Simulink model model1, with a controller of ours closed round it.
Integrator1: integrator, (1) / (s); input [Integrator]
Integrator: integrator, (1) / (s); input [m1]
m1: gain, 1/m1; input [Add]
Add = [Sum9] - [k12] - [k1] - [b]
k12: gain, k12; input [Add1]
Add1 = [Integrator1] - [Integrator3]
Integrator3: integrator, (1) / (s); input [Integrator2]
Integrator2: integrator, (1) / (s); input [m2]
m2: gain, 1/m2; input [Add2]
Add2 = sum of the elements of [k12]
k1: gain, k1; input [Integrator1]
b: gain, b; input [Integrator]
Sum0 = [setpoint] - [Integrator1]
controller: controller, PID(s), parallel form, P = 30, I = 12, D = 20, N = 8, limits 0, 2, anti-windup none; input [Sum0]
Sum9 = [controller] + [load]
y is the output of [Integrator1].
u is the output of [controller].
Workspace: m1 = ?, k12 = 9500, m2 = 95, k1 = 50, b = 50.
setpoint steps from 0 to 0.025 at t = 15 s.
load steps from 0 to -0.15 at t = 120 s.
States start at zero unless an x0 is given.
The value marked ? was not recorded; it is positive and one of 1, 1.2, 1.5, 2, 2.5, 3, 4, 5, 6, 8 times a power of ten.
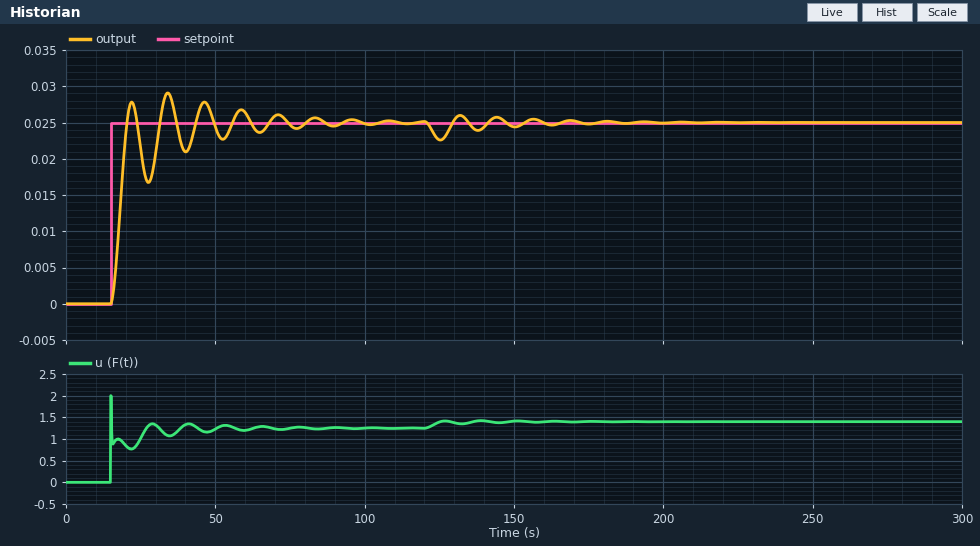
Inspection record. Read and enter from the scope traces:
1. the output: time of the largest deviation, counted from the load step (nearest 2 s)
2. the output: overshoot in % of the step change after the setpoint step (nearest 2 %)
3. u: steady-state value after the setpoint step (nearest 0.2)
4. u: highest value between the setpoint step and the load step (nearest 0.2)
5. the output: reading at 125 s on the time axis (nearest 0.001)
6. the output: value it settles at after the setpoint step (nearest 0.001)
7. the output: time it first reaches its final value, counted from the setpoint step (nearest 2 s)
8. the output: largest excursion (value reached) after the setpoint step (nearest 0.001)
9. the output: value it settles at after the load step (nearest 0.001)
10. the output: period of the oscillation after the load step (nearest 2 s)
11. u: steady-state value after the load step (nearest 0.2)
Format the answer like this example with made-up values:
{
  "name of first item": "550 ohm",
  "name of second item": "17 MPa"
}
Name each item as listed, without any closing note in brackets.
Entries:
{
  "the output: time of the largest deviation, counted from the load step": "6 s",
  "the output: overshoot in % of the step change after the setpoint step": "16 %",
  "u: steady-state value after the setpoint step": "1.2",
  "u: highest value between the setpoint step and the load step": "2.0",
  "the output: reading at 125 s on the time axis": "0.023",
  "the output: value it settles at after the setpoint step": "0.025",
  "the output: time it first reaches its final value, counted from the setpoint step": "6 s",
  "the output: largest excursion (value reached) after the setpoint step": "0.029",
  "the output: value it settles at after the load step": "0.025",
  "the output: period of the oscillation after the load step": "12 s",
  "u: steady-state value after the load step": "1.4"
}
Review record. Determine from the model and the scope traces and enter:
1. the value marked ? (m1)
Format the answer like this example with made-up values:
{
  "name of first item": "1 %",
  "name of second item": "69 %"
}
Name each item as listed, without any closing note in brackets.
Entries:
{
  "the value marked ?": "200"
}
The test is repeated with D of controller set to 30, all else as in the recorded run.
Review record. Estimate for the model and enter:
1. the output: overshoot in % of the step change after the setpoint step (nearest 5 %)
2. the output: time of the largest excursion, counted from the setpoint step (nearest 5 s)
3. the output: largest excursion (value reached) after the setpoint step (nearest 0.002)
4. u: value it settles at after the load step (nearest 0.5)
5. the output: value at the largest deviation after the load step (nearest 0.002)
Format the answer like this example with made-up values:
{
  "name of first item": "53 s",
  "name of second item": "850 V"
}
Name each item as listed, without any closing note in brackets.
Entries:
{
  "the output: overshoot in % of the step change after the setpoint step": "10 %",
  "the output: time of the largest excursion, counted from the setpoint step": "20 s",
  "the output: largest excursion (value reached) after the setpoint step": "0.028",
  "u: value it settles at after the load step": "1.5",
  "the output: value at the largest deviation after the load step": "0.022"
}
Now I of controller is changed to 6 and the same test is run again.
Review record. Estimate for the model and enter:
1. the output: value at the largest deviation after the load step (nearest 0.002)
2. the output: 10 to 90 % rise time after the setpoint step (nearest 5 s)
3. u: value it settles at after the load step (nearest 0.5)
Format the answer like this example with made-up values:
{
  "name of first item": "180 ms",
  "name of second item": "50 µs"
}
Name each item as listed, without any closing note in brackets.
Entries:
{
  "the output: value at the largest deviation after the load step": "0.022",
  "the output: 10 to 90 % rise time after the setpoint step": "15 s",
  "u: value it settles at after the load step": "1.5"
}
